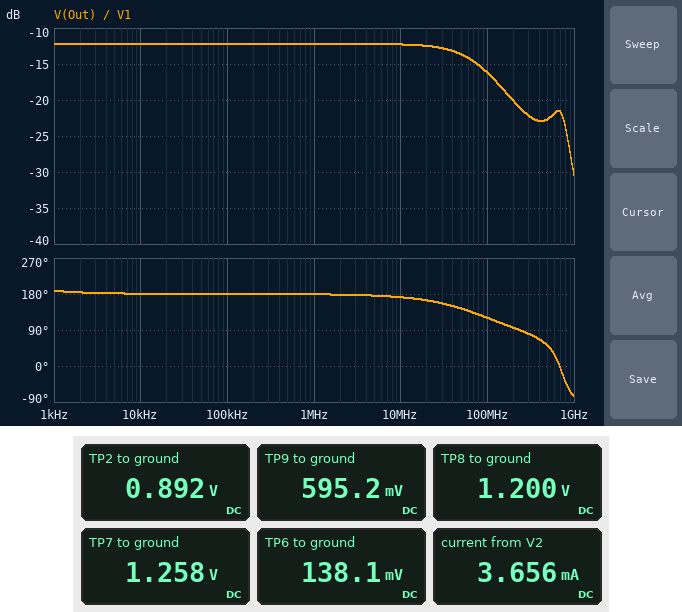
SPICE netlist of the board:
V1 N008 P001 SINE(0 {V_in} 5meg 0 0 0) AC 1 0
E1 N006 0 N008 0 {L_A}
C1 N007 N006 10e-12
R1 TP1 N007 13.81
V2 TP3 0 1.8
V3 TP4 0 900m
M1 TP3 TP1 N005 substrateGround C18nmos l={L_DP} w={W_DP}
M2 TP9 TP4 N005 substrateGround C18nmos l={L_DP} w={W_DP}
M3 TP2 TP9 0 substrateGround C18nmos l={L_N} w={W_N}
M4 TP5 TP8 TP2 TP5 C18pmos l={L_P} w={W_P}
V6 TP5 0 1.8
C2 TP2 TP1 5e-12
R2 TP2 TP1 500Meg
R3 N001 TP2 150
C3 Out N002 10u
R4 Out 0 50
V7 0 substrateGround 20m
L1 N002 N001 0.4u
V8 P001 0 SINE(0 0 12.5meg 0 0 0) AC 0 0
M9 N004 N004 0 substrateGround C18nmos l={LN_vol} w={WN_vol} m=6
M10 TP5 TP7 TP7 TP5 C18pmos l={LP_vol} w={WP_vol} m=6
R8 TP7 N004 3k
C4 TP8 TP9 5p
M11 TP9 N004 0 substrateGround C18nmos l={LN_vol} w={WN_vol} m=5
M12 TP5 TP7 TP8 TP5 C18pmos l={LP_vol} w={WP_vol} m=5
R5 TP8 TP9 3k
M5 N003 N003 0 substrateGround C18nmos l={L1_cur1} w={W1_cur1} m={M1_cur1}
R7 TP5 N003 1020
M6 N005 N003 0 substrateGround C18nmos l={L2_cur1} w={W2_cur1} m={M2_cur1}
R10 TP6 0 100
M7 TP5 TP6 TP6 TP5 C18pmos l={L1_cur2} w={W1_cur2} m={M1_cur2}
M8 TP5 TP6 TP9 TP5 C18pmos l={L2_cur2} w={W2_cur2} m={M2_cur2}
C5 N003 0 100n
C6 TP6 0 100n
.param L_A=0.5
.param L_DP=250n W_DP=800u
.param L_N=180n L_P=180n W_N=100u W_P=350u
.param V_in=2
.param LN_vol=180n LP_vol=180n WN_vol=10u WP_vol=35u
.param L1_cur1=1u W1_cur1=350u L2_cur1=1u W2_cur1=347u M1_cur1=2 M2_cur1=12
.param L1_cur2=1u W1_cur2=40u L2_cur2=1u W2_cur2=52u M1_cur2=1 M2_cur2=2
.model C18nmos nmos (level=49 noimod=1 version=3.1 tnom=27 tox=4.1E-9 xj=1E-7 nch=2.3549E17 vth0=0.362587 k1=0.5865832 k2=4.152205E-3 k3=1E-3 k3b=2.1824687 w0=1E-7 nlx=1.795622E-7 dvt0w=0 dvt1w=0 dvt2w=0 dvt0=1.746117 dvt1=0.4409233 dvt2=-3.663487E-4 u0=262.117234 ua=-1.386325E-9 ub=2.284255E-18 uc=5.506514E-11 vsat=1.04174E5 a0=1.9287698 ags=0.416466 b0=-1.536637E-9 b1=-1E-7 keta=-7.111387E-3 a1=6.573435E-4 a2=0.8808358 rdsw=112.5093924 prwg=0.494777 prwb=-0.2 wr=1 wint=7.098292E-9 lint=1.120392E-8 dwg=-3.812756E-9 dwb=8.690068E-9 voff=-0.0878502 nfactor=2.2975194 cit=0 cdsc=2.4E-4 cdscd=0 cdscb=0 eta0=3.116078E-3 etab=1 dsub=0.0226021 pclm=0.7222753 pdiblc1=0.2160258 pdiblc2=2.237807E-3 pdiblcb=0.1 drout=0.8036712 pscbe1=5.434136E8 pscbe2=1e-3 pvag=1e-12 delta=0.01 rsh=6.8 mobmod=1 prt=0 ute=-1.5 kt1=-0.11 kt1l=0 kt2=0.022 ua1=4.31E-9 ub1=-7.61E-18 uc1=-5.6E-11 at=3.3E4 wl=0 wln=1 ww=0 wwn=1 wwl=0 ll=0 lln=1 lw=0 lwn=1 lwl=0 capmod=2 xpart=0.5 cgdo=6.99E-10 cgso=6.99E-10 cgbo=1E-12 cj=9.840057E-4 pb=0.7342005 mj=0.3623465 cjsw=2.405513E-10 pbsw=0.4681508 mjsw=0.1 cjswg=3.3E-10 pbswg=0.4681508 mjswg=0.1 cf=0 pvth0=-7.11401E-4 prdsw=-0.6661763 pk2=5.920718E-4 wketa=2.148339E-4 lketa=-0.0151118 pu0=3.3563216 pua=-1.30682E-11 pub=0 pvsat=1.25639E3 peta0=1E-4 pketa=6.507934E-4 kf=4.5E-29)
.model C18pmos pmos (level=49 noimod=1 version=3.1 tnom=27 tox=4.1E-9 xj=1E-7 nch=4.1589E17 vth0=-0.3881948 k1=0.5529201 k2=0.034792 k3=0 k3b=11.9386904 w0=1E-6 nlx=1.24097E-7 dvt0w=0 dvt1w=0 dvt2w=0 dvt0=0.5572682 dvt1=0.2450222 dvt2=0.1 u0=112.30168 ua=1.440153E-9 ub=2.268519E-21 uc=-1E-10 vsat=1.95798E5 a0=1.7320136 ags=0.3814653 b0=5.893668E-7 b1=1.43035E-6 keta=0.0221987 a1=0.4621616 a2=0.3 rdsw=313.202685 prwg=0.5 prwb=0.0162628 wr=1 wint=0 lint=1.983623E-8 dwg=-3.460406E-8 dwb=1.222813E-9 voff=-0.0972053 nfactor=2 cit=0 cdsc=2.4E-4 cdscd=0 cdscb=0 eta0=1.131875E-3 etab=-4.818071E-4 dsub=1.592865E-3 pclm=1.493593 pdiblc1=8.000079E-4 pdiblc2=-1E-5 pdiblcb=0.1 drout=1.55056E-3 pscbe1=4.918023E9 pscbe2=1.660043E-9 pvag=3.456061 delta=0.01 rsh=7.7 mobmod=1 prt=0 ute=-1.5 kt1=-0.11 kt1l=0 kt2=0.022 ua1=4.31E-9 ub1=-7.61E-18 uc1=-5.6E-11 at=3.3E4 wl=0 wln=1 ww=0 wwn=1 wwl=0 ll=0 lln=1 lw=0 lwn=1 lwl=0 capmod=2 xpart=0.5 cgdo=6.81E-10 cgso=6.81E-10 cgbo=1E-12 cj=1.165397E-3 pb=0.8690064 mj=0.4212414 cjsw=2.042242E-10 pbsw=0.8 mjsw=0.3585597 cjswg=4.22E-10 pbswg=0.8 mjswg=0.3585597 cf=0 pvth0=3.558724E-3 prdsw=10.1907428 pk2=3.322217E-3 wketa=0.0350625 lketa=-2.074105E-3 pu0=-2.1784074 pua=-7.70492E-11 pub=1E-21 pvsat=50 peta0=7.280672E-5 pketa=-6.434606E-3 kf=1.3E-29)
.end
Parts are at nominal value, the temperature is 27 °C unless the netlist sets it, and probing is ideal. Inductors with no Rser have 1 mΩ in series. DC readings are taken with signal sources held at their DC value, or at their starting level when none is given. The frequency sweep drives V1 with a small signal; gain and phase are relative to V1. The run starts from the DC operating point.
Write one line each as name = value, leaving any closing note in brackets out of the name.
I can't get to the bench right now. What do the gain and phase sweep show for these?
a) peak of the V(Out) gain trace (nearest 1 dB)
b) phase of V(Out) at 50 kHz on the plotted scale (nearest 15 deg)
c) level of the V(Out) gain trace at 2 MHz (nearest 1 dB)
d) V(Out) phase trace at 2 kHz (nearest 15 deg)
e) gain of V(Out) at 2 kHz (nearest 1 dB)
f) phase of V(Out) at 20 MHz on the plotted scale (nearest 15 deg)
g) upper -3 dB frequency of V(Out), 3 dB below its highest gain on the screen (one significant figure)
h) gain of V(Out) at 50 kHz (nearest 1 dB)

peak of the V(Out) gain trace = -12 dB
phase of V(Out) at 50 kHz on the plotted scale = 180 deg
level of the V(Out) gain trace at 2 MHz = -12 dB
V(Out) phase trace at 2 kHz = 180 deg
gain of V(Out) at 2 kHz = -12 dB
phase of V(Out) at 20 MHz on the plotted scale = 165 deg
upper -3 dB frequency of V(Out), 3 dB below its highest gain on the screen = 80 MHz
gain of V(Out) at 50 kHz = -12 dB
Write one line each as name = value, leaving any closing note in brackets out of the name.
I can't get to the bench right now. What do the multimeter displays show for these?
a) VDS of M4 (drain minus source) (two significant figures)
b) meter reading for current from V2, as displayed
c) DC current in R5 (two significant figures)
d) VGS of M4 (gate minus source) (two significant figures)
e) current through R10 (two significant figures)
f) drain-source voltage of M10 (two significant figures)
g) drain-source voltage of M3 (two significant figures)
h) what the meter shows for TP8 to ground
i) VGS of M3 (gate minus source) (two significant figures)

VDS of M4 (drain minus source) = 910 mV
meter reading for current from V2, as displayed = 3.656 mA
DC current in R5 = 200 µA
VGS of M4 (gate minus source) = 310 mV
current through R10 = 1.4 mA
drain-source voltage of M10 = 540 mV
drain-source voltage of M3 = 890 mV
what the meter shows for TP8 to ground = 1.200 V
VGS of M3 (gate minus source) = 600 mV
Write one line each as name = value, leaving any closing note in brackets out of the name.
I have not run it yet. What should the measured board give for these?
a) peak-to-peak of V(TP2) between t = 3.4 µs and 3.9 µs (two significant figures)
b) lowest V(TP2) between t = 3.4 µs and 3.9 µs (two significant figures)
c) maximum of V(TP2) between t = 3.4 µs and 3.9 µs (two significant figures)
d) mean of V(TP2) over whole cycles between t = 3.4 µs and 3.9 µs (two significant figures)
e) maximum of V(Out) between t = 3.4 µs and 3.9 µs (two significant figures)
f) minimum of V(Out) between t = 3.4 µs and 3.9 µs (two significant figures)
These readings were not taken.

peak-to-peak of V(TP2) between t = 3.4 µs and 3.9 µs = 1.6 V
lowest V(TP2) between t = 3.4 µs and 3.9 µs = 84 mV
maximum of V(TP2) between t = 3.4 µs and 3.9 µs = 1.7 V
mean of V(TP2) over whole cycles between t = 3.4 µs and 3.9 µs = 880 mV
maximum of V(Out) between t = 3.4 µs and 3.9 µs = 200 mV
minimum of V(Out) between t = 3.4 µs and 3.9 µs = -200 mV
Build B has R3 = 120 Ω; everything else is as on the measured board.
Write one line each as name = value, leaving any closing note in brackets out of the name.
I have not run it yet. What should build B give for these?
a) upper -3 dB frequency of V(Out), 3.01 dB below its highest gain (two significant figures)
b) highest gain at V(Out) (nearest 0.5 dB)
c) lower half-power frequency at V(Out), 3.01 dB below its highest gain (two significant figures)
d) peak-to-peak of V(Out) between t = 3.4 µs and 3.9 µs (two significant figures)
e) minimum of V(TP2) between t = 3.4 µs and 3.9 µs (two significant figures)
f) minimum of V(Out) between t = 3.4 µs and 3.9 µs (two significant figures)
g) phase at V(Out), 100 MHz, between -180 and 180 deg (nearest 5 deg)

upper -3 dB frequency of V(Out), 3.01 dB below its highest gain = 68 MHz
highest gain at V(Out) = -11.0 dB
lower half-power frequency at V(Out), 3.01 dB below its highest gain = 120 Hz
peak-to-peak of V(Out) between t = 3.4 µs and 3.9 µs = 460 mV
minimum of V(TP2) between t = 3.4 µs and 3.9 µs = 98 mV
minimum of V(Out) between t = 3.4 µs and 3.9 µs = -230 mV
phase at V(Out), 100 MHz, between -180 and 180 deg = 115 deg
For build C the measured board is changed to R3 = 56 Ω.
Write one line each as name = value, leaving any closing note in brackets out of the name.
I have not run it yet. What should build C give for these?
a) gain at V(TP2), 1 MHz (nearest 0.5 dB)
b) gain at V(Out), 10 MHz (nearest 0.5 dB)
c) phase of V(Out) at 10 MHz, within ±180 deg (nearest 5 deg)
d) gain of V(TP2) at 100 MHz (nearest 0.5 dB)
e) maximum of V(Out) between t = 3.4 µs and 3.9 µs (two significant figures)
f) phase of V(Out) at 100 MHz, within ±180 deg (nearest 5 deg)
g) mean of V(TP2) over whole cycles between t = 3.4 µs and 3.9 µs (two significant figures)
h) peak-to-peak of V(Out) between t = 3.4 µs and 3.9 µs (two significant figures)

gain at V(TP2), 1 MHz = -0.5 dB
gain at V(Out), 10 MHz = -7.0 dB
phase of V(Out) at 10 MHz, within ±180 deg = 165 deg
gain of V(TP2) at 100 MHz = 0 dB
maximum of V(Out) between t = 3.4 µs and 3.9 µs = 330 mV
phase of V(Out) at 100 MHz, within ±180 deg = 105 deg
mean of V(TP2) over whole cycles between t = 3.4 µs and 3.9 µs = 870 mV
peak-to-peak of V(Out) between t = 3.4 µs and 3.9 µs = 680 mV
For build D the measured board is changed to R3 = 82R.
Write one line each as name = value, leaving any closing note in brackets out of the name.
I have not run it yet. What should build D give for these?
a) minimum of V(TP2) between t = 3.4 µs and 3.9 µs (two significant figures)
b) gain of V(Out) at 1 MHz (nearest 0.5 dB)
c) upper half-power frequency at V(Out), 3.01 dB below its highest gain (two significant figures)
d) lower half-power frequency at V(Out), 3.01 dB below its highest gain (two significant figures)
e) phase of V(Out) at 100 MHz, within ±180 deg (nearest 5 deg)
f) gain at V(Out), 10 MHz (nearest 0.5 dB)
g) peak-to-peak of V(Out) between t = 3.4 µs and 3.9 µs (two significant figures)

minimum of V(TP2) between t = 3.4 µs and 3.9 µs = 120 mV
gain of V(Out) at 1 MHz = -8.5 dB
upper half-power frequency at V(Out), 3.01 dB below its highest gain = 53 MHz
lower half-power frequency at V(Out), 3.01 dB below its highest gain = 140 Hz
phase of V(Out) at 100 MHz, within ±180 deg = 110 deg
gain at V(Out), 10 MHz = -9.0 dB
peak-to-peak of V(Out) between t = 3.4 µs and 3.9 µs = 570 mV
